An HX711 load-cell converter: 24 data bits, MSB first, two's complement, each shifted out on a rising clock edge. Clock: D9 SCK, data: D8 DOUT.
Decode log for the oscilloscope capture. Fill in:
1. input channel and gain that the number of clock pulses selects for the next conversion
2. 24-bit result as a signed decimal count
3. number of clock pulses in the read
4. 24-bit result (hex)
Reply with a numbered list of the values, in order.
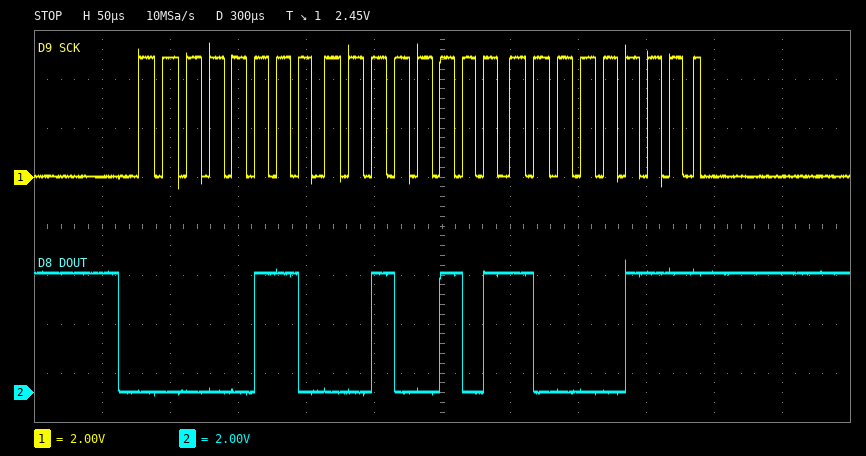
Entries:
1. channel A, gain 128
2. 402823
3. 25
4. 0x062587
